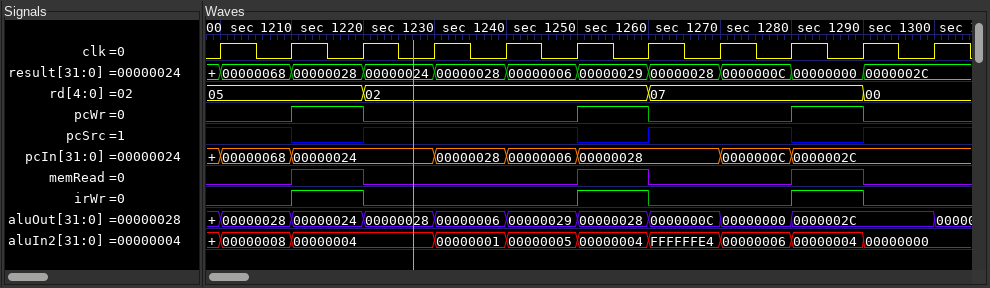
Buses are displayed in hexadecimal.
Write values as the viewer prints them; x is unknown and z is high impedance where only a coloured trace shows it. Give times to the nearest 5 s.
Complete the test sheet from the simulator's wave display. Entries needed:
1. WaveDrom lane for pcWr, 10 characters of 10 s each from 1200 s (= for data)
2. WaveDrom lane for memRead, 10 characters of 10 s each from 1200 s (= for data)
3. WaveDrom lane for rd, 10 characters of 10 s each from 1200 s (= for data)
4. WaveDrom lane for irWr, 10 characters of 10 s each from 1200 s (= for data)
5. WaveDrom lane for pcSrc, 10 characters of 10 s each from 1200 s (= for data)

{name: 'pcWr', wave: '010..10.10'}
{name: 'memRead', wave: '010..10.10'}
{name: 'rd', wave: '=.=...=..=', data: '05 02 07 00'}
{name: 'irWr', wave: '010..10.10'}
{name: 'pcSrc', wave: '101..01.01'}
